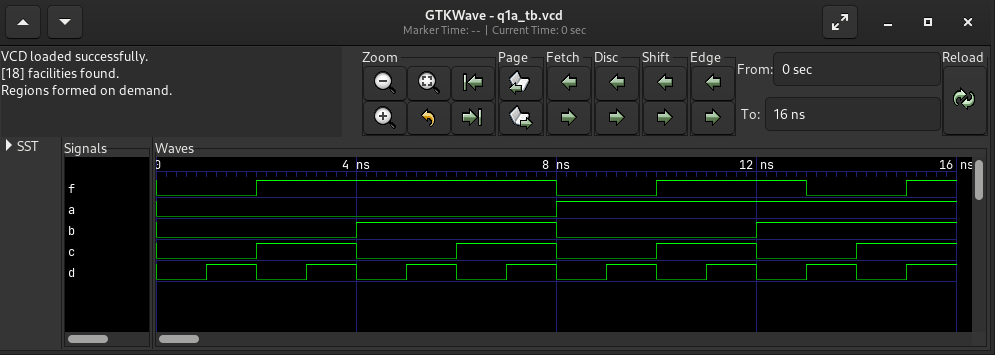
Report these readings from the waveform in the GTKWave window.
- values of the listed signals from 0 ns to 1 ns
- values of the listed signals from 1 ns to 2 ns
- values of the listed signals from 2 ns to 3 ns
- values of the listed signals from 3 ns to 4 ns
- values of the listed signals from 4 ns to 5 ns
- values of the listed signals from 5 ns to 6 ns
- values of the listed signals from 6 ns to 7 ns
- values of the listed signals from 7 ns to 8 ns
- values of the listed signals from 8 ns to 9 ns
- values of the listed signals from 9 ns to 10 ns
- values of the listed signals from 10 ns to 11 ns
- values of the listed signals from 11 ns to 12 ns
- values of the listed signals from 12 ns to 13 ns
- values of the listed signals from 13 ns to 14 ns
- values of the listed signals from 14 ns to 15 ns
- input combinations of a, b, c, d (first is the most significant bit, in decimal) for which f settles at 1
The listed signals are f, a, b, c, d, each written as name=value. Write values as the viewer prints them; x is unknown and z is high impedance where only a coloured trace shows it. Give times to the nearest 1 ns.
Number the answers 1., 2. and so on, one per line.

1. f=0, a=0, b=0, c=0, d=0
2. f=0, a=0, b=0, c=0, d=1
3. f=1, a=0, b=0, c=1, d=0
4. f=1, a=0, b=0, c=1, d=1
5. f=1, a=0, b=1, c=0, d=0
6. f=1, a=0, b=1, c=0, d=1
7. f=1, a=0, b=1, c=1, d=0
8. f=1, a=0, b=1, c=1, d=1
9. f=0, a=1, b=0, c=0, d=0
10. f=0, a=1, b=0, c=0, d=1
11. f=1, a=1, b=0, c=1, d=0
12. f=1, a=1, b=0, c=1, d=1
13. f=1, a=1, b=1, c=0, d=0
14. f=0, a=1, b=1, c=0, d=1
15. f=0, a=1, b=1, c=1, d=0
16. 2, 3, 4, 5, 6, 7, 10, 11, 12, 15
